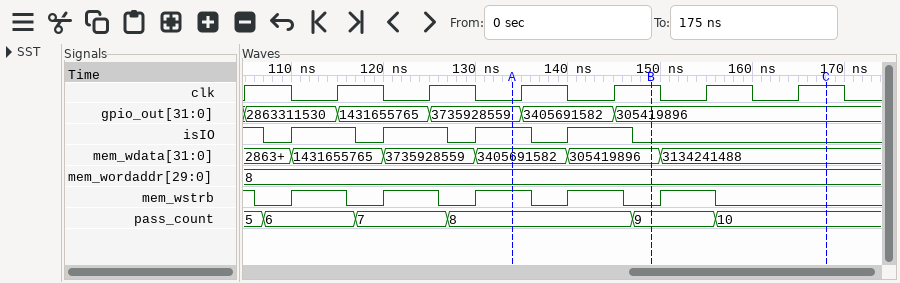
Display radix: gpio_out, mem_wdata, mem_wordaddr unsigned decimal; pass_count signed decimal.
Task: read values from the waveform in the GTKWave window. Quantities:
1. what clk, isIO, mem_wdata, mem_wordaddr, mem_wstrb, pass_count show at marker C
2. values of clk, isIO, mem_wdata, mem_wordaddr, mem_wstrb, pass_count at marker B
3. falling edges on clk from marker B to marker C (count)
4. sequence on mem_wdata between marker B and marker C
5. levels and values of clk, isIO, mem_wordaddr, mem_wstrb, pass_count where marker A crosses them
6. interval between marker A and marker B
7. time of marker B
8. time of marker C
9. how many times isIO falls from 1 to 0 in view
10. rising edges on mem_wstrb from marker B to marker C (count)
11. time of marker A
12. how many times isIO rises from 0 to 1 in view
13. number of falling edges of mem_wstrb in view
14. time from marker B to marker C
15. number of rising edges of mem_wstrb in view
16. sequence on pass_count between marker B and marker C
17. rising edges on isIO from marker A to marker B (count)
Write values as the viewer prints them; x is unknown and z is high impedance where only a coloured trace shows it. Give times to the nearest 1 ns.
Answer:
clk=1, isIO=0, mem_wdata=3134241488, mem_wordaddr=8, mem_wstrb=0, pass_count=10
clk=1, isIO=0, mem_wdata=305419896, mem_wordaddr=8, mem_wstrb=0, pass_count=9
2
305419896, 3134241488
clk=0, isIO=1, mem_wordaddr=8, mem_wstrb=1, pass_count=8
15 ns
149 ns
168 ns
5
1
134 ns
4
6
19 ns
5
9, 10
1
